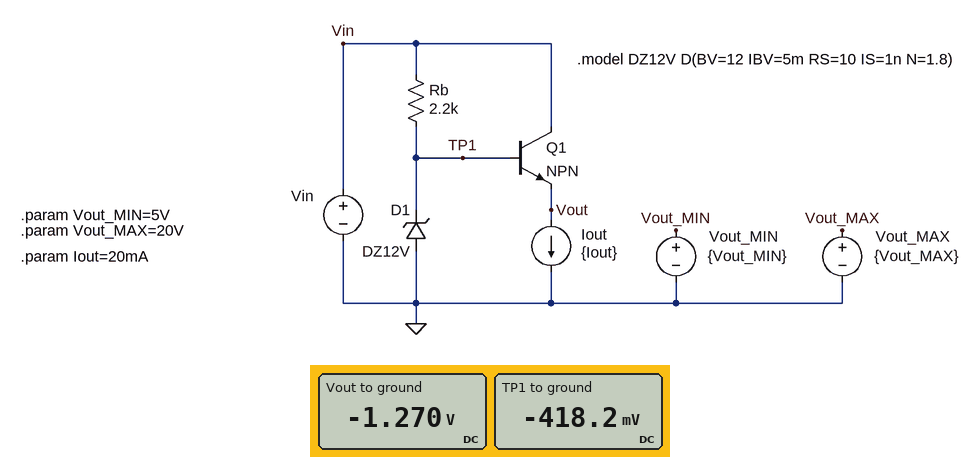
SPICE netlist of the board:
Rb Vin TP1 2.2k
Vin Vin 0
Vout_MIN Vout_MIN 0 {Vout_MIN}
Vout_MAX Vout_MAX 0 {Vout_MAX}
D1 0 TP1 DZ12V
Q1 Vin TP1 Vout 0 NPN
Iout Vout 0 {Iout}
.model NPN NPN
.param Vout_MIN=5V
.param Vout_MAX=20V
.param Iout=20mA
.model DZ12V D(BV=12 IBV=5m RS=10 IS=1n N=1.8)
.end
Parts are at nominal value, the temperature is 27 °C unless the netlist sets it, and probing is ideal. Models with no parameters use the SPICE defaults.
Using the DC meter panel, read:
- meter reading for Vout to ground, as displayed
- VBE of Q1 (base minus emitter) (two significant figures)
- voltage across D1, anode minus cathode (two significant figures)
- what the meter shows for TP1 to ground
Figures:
-1.270 V
850 mV
420 mV
-418.2 mV
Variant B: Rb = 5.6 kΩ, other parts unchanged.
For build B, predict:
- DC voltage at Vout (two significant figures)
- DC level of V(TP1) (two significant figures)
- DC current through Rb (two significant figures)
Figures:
-1.4 V
-540 mV
96 µA
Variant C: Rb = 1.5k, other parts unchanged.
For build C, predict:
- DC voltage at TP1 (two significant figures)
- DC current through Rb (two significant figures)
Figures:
-300 mV
200 µA
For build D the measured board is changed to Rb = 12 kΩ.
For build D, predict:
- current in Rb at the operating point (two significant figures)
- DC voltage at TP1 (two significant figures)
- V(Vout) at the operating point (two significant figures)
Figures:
46 µA
-560 mV
-1.4 V
